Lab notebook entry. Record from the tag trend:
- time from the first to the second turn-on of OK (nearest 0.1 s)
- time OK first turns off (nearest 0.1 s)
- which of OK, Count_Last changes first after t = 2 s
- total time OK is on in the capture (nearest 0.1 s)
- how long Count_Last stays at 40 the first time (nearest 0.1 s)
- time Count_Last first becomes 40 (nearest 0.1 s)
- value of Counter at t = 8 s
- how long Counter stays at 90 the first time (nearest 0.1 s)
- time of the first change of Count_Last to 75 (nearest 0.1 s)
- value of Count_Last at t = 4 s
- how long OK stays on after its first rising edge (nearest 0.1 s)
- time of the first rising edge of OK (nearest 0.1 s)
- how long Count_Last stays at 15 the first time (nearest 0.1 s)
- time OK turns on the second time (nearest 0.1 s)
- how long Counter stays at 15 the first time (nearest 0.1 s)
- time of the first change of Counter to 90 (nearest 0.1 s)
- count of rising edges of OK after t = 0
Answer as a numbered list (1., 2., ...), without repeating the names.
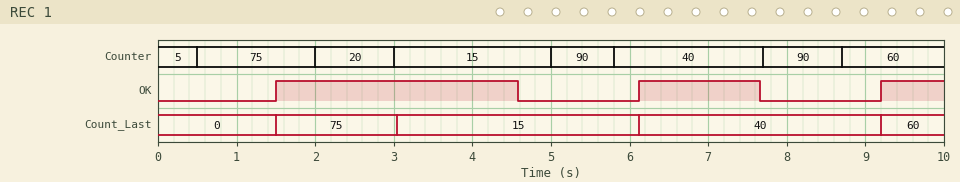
1. 4.6 s
2. 4.6 s
3. Count_Last
4. 5.4 s
5. 3.1 s
6. 6.1 s
7. 90
8. 0.8 s
9. 1.5 s
10. 15
11. 3.1 s
12. 1.5 s
13. 3.1 s
14. 6.1 s
15. 2.0 s
16. 5.0 s
17. 3
